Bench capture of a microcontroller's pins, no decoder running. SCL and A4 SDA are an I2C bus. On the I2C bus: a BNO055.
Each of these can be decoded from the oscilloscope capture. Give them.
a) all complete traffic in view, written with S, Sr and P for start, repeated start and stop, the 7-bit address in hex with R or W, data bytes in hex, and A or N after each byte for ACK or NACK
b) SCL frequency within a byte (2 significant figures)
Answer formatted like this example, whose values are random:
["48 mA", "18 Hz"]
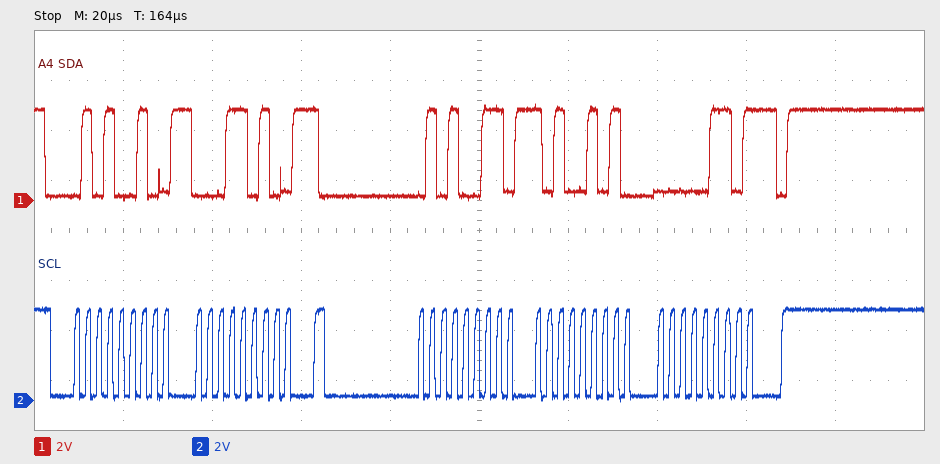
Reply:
["S 29W A 1A A Sr 29R A A5 A 06 N P", "400 kHz"]
